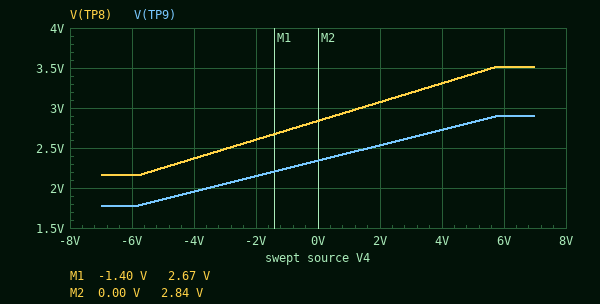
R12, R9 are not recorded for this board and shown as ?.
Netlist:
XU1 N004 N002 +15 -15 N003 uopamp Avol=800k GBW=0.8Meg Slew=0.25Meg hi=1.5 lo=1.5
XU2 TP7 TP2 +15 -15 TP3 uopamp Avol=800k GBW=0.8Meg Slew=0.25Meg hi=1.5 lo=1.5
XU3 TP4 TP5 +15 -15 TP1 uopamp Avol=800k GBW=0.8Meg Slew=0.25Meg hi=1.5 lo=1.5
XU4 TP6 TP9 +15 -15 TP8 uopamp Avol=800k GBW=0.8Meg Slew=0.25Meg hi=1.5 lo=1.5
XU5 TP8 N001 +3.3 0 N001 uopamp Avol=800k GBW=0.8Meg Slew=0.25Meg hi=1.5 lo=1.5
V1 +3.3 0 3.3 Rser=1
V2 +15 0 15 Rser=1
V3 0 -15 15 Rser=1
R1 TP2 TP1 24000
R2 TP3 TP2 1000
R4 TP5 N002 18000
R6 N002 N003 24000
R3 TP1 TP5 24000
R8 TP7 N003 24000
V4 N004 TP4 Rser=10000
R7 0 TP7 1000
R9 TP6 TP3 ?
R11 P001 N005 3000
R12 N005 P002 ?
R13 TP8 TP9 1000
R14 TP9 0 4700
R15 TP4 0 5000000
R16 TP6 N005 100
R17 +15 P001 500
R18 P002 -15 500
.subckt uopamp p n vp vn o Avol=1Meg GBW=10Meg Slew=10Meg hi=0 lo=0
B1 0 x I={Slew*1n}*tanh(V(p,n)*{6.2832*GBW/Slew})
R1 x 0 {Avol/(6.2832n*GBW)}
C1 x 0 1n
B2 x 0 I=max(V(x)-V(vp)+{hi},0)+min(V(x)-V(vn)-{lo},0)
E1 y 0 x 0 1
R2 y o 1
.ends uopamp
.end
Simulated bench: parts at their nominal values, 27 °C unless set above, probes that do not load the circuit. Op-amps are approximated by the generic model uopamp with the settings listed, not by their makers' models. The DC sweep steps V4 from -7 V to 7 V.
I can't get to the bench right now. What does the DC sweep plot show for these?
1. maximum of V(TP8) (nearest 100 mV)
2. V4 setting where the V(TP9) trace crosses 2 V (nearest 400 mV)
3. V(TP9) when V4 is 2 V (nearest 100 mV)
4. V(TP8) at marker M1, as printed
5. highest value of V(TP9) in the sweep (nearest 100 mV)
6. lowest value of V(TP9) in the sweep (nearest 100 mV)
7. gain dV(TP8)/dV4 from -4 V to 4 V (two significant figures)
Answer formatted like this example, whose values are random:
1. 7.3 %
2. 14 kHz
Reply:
1. 3.5 V
2. -3.6 V
3. 2.5 V
4. 2.67 V
5. 2.9 V
6. 1.8 V
7. 0.12 V/V
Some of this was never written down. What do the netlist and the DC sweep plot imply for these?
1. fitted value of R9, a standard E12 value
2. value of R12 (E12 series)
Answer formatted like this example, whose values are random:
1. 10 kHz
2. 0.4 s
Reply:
1. 1.5 kΩ
2. 8.2 kΩ
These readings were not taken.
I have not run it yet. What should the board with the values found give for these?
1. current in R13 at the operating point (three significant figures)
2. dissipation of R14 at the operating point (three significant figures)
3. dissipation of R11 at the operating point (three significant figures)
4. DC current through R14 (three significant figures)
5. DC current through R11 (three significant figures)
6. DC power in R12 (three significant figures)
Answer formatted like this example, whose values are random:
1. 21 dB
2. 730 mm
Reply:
1. 498 µA
2. 1.17 mW
3. 38.3 mW
4. 498 µA
5. 3.57 mA
6. 33.2 mW
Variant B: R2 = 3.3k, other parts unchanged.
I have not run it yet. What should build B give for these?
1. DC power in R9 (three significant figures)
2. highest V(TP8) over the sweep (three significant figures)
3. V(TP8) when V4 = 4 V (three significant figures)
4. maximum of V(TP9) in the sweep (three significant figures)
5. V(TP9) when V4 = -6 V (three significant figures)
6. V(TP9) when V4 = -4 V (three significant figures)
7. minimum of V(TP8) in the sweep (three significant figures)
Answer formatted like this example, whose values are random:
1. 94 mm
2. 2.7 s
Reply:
1. 3.65 mW
2. 4.13 V
3. 3.73 V
4. 3.40 V
5. 1.28 V
6. 1.61 V
7. 1.55 V
